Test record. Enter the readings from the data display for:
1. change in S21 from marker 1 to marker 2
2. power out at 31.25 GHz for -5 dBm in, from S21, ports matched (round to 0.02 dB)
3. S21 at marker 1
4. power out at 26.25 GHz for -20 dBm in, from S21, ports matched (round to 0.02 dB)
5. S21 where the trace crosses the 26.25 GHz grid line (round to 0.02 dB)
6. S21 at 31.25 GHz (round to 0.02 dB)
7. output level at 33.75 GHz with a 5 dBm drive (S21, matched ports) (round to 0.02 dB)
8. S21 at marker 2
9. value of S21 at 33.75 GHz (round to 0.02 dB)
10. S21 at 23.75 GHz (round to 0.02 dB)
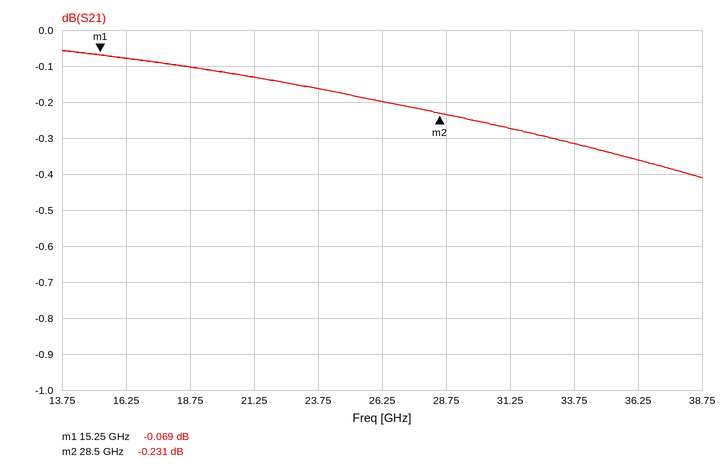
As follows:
-0.162 dB
-5.28 dBm
-0.069 dB
-20.20 dBm
-0.20 dB
-0.28 dB
4.68 dBm
-0.231 dB
-0.32 dB
-0.16 dB
